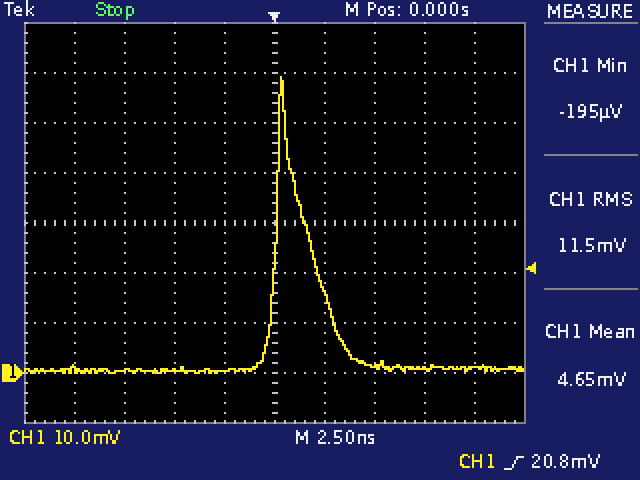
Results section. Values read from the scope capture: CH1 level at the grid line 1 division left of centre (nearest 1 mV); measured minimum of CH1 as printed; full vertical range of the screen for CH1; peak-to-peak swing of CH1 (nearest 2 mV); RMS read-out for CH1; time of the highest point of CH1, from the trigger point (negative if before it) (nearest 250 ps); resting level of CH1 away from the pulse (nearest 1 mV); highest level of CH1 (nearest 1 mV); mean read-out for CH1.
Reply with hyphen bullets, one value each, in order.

- 0 mV
- -195 µV
- 80 mV
- 60 mV
- 11.5 mV
- +500 ps
- 1 mV
- 59 mV
- 4.65 mV
